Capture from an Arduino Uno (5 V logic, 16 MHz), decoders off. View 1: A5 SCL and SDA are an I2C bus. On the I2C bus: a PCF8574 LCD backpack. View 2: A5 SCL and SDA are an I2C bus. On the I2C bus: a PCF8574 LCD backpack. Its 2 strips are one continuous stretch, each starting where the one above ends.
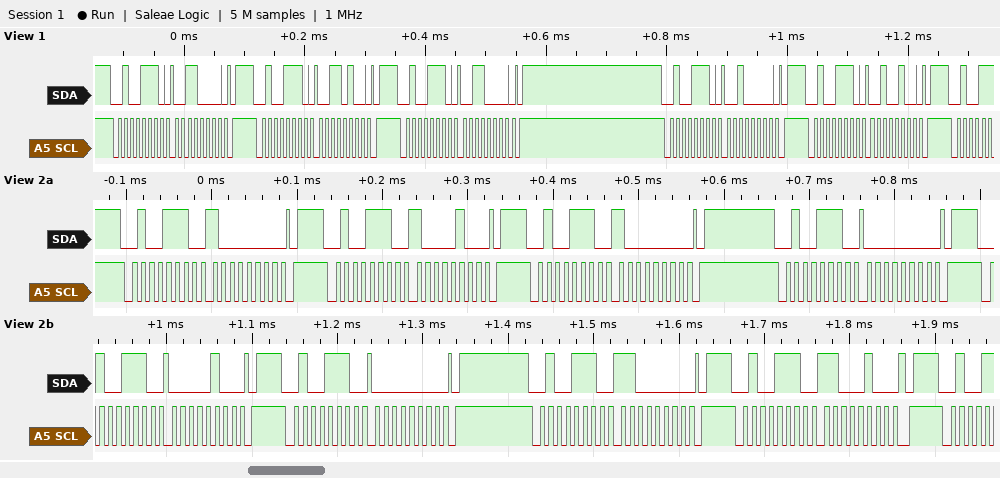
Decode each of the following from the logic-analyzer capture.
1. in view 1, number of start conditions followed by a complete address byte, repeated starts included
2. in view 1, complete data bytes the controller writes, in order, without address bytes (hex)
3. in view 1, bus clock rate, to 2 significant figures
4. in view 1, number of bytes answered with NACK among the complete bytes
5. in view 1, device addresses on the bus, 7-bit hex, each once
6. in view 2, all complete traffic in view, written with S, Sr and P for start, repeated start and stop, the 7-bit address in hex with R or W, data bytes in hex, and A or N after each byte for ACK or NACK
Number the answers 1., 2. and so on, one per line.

1. 5
2. 30 34 30 20 24
3. 100 kHz
4. 0
5. 0x27
6. S 27W A 80 A P S 27W A 84 A P S 27W A 80 A P S 27W A 00 A P S 27W A 04 A P S 27W A 00 A P S 27W A C0 A P S 27W A C4 A P
